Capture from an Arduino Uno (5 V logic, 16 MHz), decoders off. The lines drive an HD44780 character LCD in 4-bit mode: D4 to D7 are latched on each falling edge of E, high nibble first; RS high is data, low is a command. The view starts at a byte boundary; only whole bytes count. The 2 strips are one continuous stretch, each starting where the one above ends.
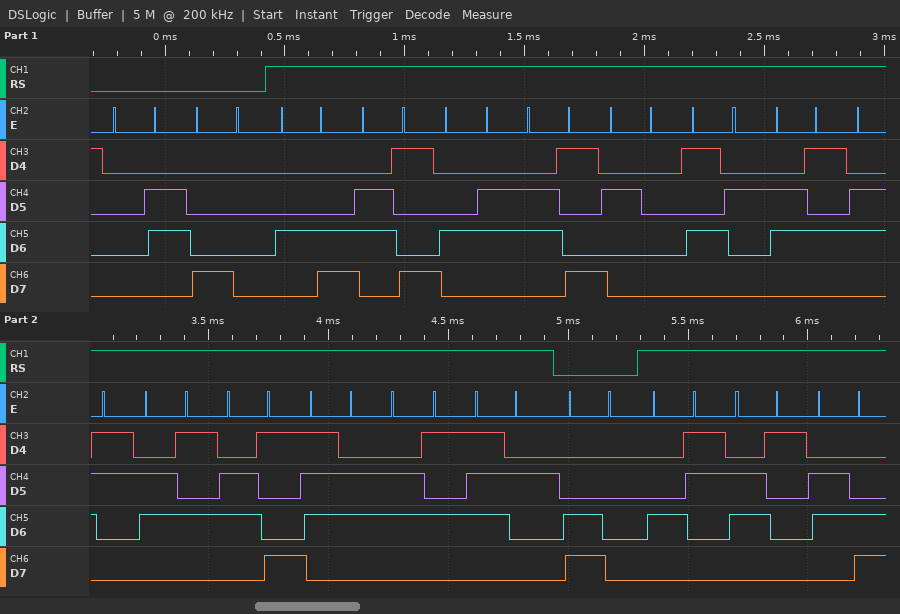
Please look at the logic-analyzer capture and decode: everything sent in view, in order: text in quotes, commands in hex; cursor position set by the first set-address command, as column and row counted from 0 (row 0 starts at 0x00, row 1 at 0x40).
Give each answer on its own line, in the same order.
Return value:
0x06 0x80 "LiFi Receiver" 0xC0 "Cal"
column 0, row 0
